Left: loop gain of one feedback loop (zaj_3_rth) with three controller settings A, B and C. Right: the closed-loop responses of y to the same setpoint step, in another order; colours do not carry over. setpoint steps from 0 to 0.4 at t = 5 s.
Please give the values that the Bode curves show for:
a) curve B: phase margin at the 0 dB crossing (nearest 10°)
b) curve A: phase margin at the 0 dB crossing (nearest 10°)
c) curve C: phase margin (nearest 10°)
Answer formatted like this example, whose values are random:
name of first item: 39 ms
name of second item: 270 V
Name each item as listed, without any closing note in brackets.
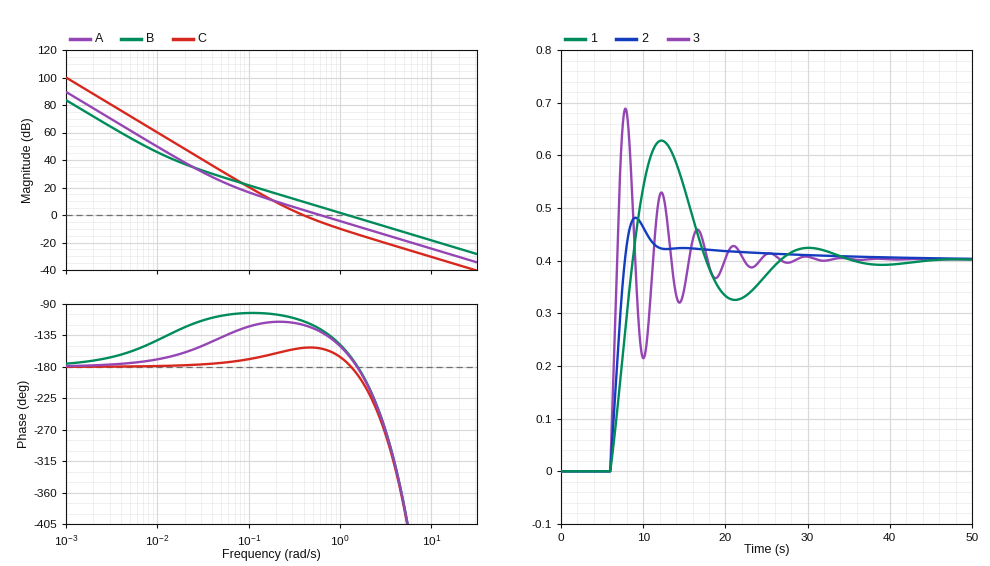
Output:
curve B: phase margin at the 0 dB crossing: 20°
curve A: phase margin at the 0 dB crossing: 50°
curve C: phase margin: 30°
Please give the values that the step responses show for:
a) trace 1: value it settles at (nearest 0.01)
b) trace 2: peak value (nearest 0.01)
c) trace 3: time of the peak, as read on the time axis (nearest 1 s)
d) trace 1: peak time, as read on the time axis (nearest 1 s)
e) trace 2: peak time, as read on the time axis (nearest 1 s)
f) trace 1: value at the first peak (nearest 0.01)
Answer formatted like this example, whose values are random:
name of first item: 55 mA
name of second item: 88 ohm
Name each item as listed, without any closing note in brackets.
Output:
trace 1: value it settles at: 0.40
trace 2: peak value: 0.48
trace 3: time of the peak, as read on the time axis: 8 s
trace 1: peak time, as read on the time axis: 12 s
trace 2: peak time, as read on the time axis: 9 s
trace 1: value at the first peak: 0.63
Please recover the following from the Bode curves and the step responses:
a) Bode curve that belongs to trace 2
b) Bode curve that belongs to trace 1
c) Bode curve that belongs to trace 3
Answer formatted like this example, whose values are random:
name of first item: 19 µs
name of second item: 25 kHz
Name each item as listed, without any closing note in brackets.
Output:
Bode curve that belongs to trace 2: A
Bode curve that belongs to trace 1: C
Bode curve that belongs to trace 3: B
